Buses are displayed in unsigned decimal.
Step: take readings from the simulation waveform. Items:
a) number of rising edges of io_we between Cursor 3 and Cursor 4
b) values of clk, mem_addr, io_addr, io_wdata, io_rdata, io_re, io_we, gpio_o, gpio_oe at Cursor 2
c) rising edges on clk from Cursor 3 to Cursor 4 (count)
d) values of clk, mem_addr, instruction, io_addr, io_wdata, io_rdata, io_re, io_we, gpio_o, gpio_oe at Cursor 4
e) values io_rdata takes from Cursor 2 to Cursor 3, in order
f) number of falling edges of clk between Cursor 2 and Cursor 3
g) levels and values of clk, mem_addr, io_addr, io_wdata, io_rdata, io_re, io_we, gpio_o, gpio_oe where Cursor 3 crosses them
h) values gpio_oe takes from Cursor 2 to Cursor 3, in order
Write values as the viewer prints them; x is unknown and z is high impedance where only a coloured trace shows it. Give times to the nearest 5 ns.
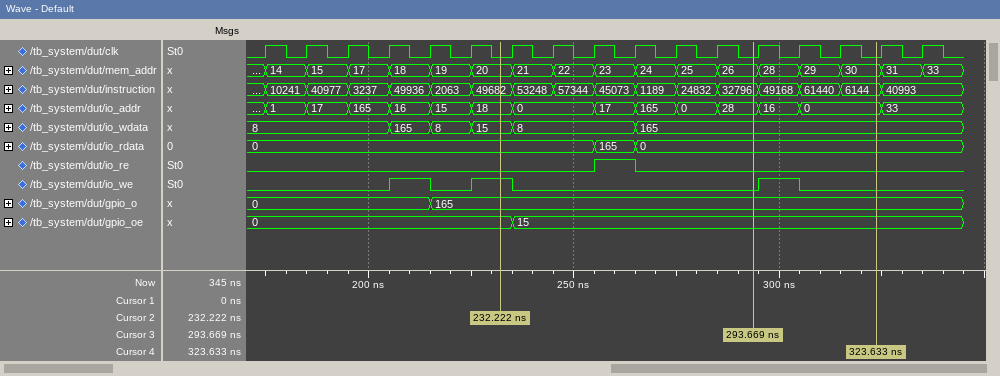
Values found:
1
clk=0, mem_addr=20, io_addr=18, io_wdata=15, io_rdata=0, io_re=0, io_we=1, gpio_o=165, gpio_oe=0
3
clk=0, mem_addr=30, instruction=6144, io_addr=0, io_wdata=165, io_rdata=0, io_re=0, io_we=0, gpio_o=165, gpio_oe=15
0, 165, 0
6
clk=0, mem_addr=26, io_addr=28, io_wdata=165, io_rdata=0, io_re=0, io_we=0, gpio_o=165, gpio_oe=15
0, 15
